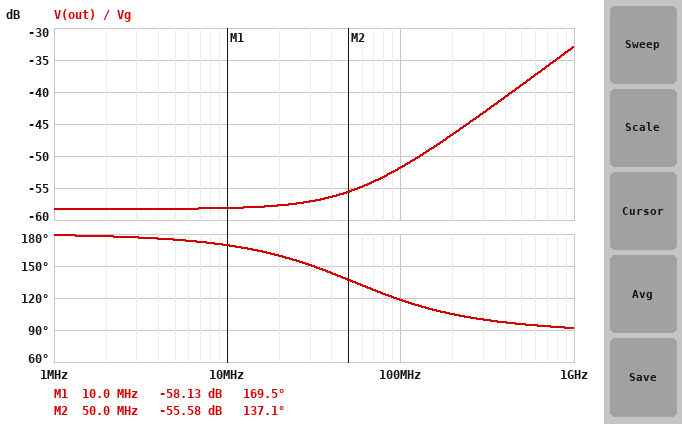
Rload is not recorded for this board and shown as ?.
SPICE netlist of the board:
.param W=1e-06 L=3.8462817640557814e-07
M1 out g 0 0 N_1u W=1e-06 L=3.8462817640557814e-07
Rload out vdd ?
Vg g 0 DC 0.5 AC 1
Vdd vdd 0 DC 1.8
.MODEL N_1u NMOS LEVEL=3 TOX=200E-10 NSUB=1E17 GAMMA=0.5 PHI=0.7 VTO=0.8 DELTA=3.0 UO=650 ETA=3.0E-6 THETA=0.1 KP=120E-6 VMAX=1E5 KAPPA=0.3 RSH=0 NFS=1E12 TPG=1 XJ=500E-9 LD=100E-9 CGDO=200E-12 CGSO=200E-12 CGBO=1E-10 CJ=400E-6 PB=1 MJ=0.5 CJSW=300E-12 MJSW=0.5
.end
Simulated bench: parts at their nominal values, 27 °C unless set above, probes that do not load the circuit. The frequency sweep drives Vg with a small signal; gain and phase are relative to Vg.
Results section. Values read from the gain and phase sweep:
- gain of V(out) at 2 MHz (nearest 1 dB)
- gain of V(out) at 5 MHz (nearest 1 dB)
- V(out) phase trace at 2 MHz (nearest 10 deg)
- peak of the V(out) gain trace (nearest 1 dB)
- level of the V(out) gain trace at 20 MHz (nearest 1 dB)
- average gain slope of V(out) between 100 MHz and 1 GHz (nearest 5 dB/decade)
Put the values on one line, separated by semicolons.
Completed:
-58 dB; -58 dB; 180 deg; -33 dB; -58 dB; 20 dB/decade
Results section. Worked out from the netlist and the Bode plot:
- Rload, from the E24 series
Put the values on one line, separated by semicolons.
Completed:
18 kΩ
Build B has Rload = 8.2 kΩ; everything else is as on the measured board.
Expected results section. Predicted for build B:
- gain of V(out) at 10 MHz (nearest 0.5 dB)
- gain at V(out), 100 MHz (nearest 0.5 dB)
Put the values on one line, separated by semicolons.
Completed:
-65.0 dB; -58.5 dB
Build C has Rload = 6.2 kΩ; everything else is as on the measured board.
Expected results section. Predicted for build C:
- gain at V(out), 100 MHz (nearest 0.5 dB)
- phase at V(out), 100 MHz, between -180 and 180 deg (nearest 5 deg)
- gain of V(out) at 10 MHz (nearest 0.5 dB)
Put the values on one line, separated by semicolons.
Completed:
-61.0 dB; 120 deg; -67.5 dB
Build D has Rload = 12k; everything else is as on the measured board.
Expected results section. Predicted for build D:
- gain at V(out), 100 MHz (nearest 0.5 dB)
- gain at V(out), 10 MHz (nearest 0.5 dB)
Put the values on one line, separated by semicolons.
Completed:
-55.5 dB; -61.5 dB
